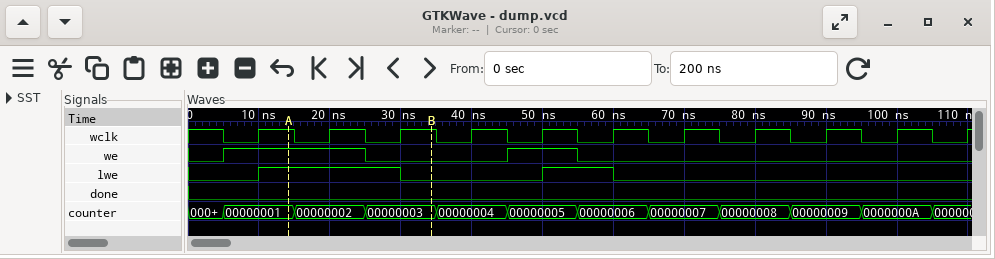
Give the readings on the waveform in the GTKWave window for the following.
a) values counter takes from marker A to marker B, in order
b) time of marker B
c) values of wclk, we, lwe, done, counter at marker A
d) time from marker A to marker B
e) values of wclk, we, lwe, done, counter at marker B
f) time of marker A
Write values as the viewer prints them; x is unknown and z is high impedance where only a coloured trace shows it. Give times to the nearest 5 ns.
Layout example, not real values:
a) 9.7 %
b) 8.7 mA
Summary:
a) 00000001, 00000002, 00000003
b) 35 ns
c) wclk=1, we=1, lwe=1, done=0, counter=00000001
d) 20 ns
e) wclk=1, we=0, lwe=0, done=0, counter=00000003
f) 15 ns
